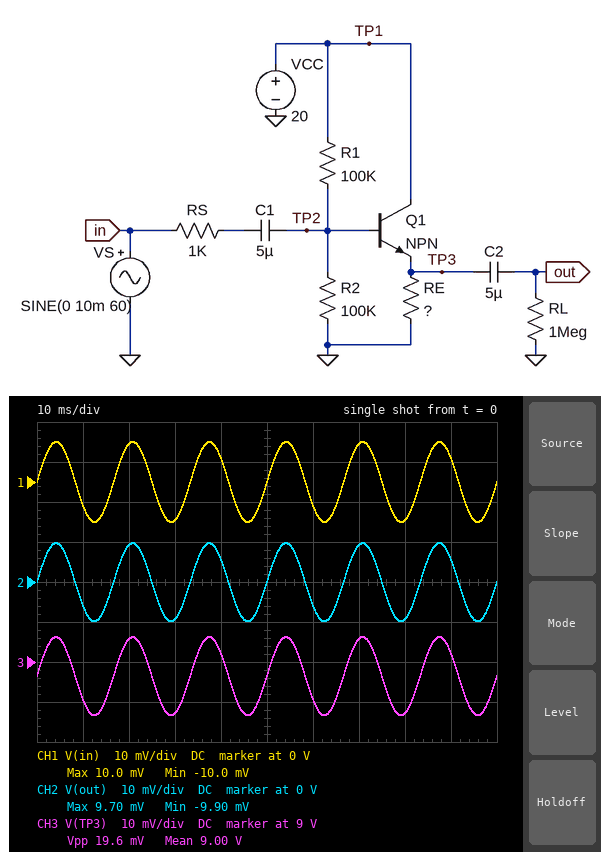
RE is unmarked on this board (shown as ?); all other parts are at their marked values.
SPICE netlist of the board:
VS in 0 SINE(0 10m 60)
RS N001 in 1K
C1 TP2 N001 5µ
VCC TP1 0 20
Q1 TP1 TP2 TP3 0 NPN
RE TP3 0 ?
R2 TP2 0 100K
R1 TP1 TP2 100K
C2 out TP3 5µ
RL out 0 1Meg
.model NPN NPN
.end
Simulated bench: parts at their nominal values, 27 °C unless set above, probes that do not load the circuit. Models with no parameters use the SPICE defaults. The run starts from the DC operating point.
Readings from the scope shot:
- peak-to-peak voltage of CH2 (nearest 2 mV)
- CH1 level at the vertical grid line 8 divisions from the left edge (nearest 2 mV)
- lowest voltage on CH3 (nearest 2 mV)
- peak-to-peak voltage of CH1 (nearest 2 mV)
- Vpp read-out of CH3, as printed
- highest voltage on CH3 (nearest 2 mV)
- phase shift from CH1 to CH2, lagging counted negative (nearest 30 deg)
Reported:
20 mV
-10 mV
8.986 V
20 mV
19.6 mV
9.006 V
0 deg
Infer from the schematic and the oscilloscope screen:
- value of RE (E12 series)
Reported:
18 kΩ
